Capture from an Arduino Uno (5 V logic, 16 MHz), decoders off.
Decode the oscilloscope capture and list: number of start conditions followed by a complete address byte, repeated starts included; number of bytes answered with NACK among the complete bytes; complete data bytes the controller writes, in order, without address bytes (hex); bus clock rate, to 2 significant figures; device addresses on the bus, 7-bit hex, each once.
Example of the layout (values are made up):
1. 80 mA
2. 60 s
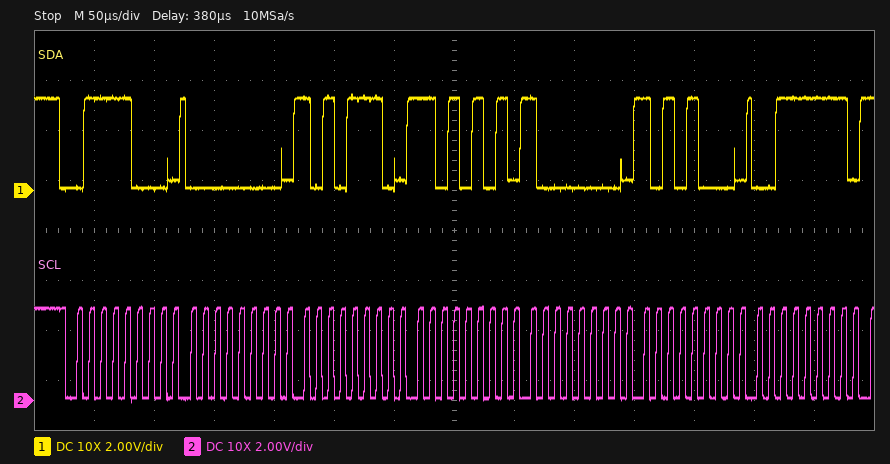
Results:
1. 1
2. 0
3. 00 AE D5 80 A8 3F
4. 100 kHz
5. 0x3C
